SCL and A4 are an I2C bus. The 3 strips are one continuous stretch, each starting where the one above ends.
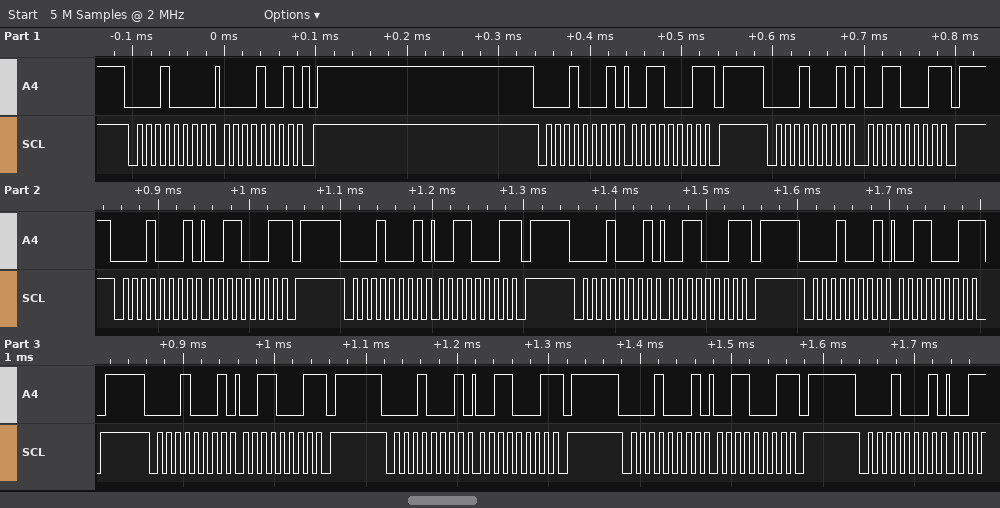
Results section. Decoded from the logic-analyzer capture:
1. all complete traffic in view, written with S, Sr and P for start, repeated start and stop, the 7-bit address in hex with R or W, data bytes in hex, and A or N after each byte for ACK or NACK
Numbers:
S 08W A 09 A P S 08R A 31 N P S 08R A 31 N P S 08R A 31 N P S 08R A 31 N P S 08R A 31 N P S 08R A 31 N P S 08R A 31 N P S 08R A 31 N P S 08R A 31 N P S 08R A
